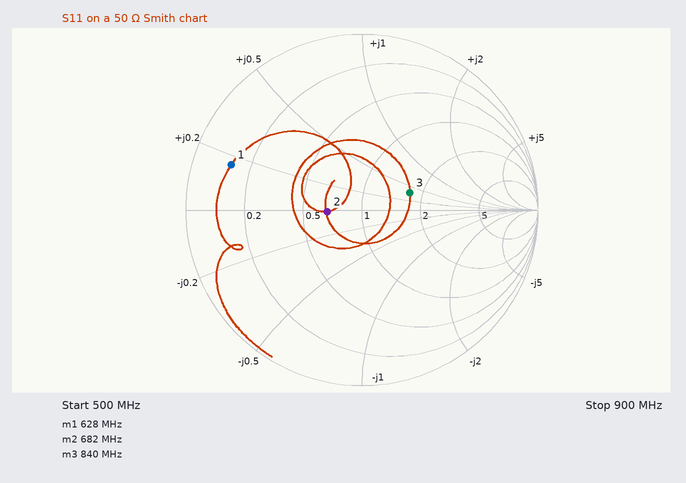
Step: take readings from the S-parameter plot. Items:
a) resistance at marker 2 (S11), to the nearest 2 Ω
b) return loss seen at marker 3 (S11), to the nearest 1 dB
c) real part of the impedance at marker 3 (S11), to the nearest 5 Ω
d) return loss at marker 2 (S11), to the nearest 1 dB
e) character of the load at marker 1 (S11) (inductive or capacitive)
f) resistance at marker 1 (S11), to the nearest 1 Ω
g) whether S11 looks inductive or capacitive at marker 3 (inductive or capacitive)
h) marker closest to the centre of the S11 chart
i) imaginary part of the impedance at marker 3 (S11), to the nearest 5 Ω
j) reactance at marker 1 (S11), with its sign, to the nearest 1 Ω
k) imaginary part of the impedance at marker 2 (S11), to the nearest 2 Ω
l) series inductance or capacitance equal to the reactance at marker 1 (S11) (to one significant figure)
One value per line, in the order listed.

34 Ω
11 dB
85 Ω
14 dB
inductive
6 Ω
inductive
marker 2
+20 Ω
+8 Ω
0 Ω
2 nH
